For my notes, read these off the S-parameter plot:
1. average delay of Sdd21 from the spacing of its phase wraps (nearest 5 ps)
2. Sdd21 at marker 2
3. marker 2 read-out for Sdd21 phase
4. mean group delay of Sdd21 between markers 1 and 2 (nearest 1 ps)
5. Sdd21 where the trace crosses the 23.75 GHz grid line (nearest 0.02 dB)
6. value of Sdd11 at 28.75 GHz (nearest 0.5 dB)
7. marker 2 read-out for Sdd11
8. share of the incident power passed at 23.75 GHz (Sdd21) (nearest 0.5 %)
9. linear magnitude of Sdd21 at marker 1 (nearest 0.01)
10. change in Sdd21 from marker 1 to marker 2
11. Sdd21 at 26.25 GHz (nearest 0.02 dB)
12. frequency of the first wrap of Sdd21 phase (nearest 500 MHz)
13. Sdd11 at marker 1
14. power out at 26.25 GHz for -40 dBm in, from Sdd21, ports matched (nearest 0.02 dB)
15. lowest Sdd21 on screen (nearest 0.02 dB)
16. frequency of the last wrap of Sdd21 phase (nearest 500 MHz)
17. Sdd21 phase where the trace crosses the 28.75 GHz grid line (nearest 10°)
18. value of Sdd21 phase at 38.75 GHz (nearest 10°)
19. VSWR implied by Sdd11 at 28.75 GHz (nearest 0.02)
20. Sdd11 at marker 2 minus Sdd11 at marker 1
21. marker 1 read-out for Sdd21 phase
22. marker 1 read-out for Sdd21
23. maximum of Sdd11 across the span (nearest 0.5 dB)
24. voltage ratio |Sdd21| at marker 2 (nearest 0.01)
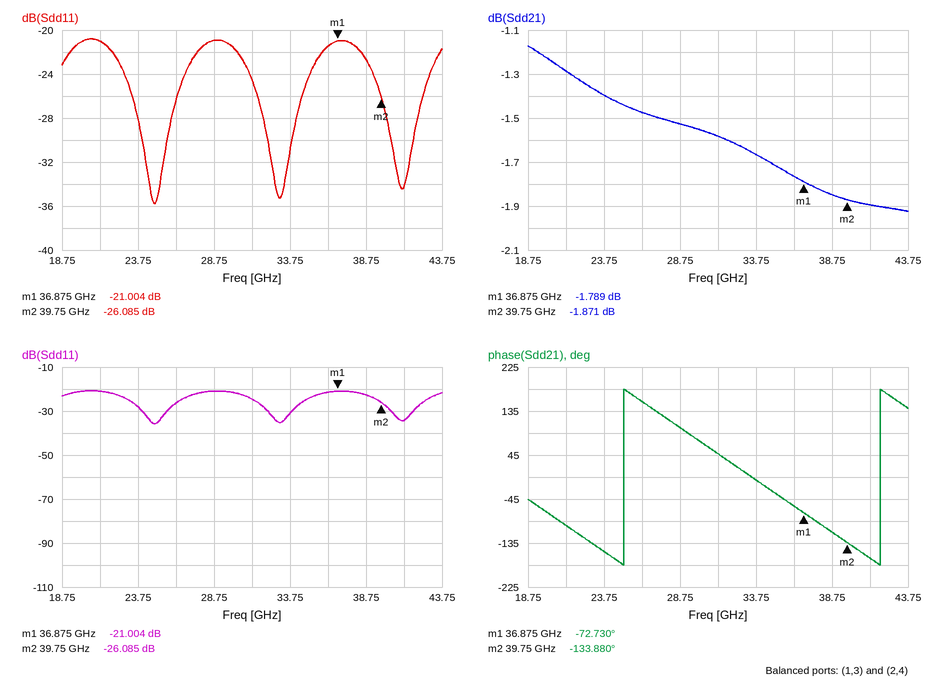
60 ps
-1.871 dB
-133.880°
59 ps
-1.40 dB
-21.0 dB
-26.085 dB
72.5 %
0.81
-0.082 dB
-1.48 dB
25.0 GHz
-21.004 dB
-41.48 dBm
-1.92 dB
42.0 GHz
100°
-110°
1.20
-5.081 dB
-72.730°
-1.789 dB
-21.0 dB
0.81
